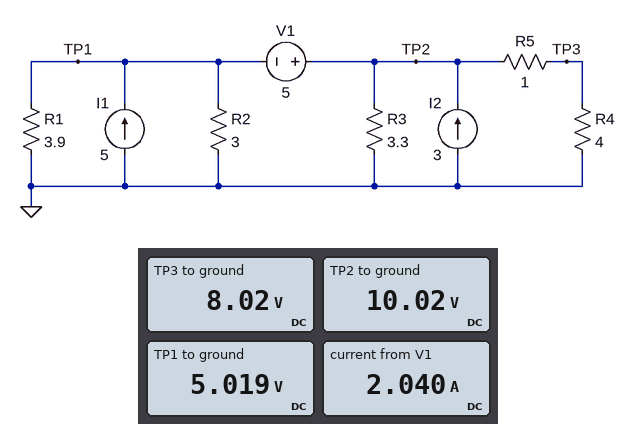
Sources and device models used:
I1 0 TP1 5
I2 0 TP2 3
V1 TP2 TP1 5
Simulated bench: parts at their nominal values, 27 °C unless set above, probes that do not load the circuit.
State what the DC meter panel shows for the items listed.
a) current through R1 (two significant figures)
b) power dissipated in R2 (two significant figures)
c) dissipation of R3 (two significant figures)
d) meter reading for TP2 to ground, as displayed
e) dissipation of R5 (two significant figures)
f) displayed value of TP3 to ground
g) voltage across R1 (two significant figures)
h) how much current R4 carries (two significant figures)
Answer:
1.3 A
8.4 W
30 W
10.02 V
4.0 W
8.02 V
5.0 V
2.0 A
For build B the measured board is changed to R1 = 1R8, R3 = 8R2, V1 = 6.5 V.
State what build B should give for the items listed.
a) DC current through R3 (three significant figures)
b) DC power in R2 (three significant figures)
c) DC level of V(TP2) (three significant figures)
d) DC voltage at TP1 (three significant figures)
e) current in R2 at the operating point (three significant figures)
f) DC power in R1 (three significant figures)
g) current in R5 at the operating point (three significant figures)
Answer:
1.39 A
7.93 W
11.4 V
4.88 V
1.63 A
13.2 W
2.28 A
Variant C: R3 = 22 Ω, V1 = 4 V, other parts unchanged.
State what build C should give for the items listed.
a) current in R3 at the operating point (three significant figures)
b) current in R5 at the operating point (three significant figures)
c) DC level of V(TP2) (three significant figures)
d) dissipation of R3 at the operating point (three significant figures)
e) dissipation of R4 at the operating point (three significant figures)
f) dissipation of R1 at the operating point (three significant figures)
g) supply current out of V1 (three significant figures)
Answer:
564 mA
2.48 A
12.4 V
6.99 W
24.6 W
18.1 W
44.4 mA
